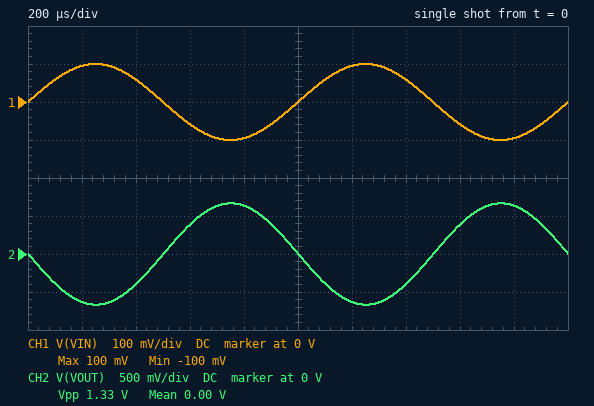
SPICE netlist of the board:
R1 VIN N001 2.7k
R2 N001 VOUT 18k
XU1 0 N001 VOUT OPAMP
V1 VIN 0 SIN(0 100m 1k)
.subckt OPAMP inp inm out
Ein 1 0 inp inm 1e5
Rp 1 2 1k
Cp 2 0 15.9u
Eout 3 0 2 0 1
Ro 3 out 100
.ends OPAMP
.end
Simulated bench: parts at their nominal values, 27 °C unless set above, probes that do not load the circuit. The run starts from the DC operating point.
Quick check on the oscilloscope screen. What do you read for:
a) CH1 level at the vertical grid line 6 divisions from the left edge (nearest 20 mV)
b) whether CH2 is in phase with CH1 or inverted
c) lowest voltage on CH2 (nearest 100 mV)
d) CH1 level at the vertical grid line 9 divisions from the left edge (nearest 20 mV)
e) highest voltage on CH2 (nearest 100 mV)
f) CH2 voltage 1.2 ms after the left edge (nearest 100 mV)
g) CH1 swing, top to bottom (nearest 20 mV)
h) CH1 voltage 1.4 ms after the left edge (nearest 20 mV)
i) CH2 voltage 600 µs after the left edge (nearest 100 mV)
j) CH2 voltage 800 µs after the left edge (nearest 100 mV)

100 mV
inverted
-700 mV
-100 mV
700 mV
-600 mV
200 mV
60 mV
400 mV
600 mV
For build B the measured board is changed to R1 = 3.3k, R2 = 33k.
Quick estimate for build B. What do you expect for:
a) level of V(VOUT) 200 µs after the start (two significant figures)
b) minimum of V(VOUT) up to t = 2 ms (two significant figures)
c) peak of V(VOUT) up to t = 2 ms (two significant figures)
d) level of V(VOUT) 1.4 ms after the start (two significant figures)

-950 mV
-1.0 V
1.0 V
-600 mV
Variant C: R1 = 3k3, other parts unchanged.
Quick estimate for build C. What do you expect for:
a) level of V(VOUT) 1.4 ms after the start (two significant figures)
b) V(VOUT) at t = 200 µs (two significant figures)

-320 mV
-520 mV
